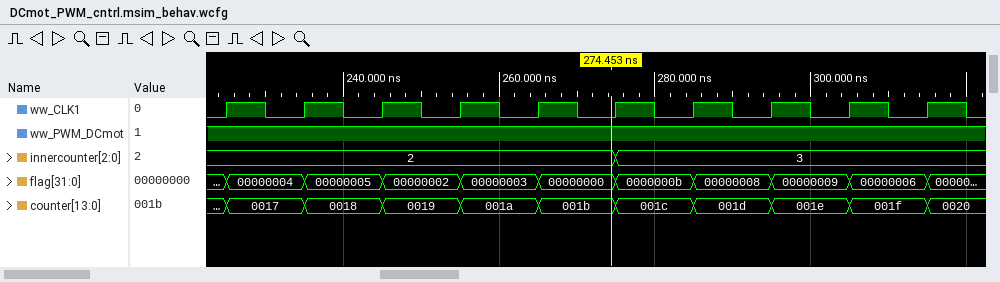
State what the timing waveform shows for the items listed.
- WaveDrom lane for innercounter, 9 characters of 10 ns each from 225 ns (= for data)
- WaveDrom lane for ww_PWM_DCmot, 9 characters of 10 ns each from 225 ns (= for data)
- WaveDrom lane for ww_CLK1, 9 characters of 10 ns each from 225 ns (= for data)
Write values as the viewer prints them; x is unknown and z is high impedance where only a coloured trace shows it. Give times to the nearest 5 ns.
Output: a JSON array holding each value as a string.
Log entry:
["{name: 'innercounter', wave: '=....=...', data: '2 3'}", "{name: 'ww_PWM_DCmot', wave: '1........'}", "{name: 'ww_CLK1', wave: 'p........'}"]
